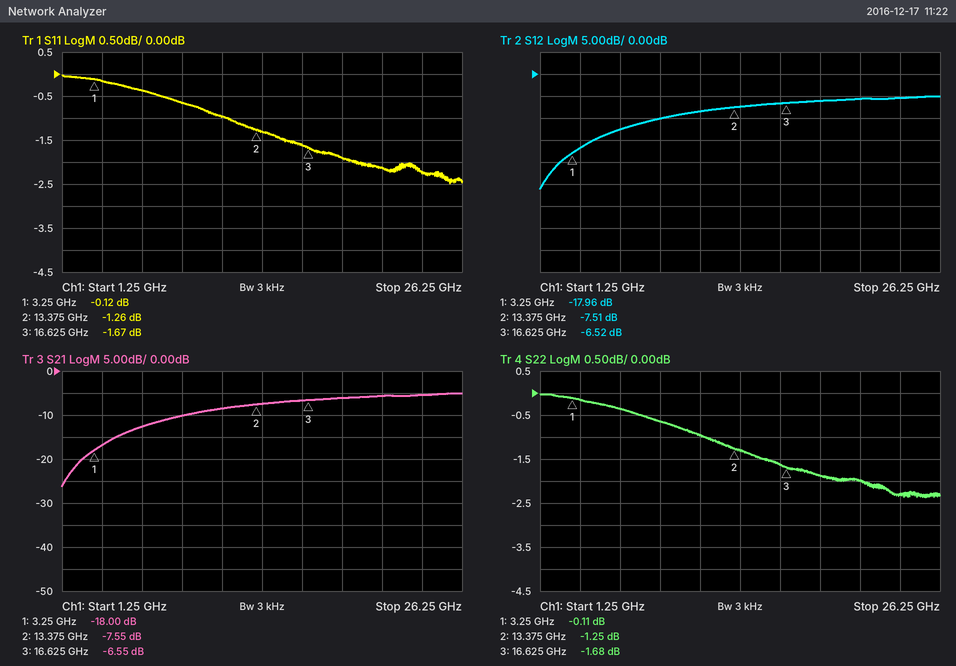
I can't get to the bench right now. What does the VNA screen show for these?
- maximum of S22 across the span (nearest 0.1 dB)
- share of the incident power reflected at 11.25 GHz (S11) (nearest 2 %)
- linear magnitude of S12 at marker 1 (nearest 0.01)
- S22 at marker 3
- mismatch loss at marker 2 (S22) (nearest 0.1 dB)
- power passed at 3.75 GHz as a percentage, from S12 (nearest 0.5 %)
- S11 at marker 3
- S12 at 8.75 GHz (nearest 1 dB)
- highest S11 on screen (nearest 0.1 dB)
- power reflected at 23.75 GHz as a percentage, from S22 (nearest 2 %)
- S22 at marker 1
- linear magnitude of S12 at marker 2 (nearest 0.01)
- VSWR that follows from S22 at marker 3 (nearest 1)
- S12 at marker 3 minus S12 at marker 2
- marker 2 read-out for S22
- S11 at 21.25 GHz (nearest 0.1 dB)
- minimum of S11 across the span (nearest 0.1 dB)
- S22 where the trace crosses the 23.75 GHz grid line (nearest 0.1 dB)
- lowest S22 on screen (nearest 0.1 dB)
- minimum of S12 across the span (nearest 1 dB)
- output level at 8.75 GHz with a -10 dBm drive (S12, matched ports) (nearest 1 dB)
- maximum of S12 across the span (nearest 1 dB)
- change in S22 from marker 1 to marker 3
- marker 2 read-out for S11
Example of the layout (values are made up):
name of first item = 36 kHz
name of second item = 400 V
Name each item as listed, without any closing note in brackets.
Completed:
maximum of S22 across the span = 0.0 dB
share of the incident power reflected at 11.25 GHz (S11) = 80 %
linear magnitude of S12 at marker 1 = 0.13
S22 at marker 3 = -1.68 dB
mismatch loss at marker 2 (S22) = 6.0 dB
power passed at 3.75 GHz as a percentage, from S12 = 2.0 %
S11 at marker 3 = -1.67 dB
S12 at 8.75 GHz = -10 dB
highest S11 on screen = 0.0 dB
power reflected at 23.75 GHz as a percentage, from S22 = 58 %
S22 at marker 1 = -0.11 dB
linear magnitude of S12 at marker 2 = 0.42
VSWR that follows from S22 at marker 3 = 10
S12 at marker 3 minus S12 at marker 2 = 0.99 dB
marker 2 read-out for S22 = -1.25 dB
S11 at 21.25 GHz = -2.1 dB
minimum of S11 across the span = -2.5 dB
S22 where the trace crosses the 23.75 GHz grid line = -2.3 dB
lowest S22 on screen = -2.4 dB
minimum of S12 across the span = -26 dB
output level at 8.75 GHz with a -10 dBm drive (S12, matched ports) = -20 dBm
maximum of S12 across the span = -5 dB
change in S22 from marker 1 to marker 3 = -1.57 dB
marker 2 read-out for S11 = -1.26 dB
